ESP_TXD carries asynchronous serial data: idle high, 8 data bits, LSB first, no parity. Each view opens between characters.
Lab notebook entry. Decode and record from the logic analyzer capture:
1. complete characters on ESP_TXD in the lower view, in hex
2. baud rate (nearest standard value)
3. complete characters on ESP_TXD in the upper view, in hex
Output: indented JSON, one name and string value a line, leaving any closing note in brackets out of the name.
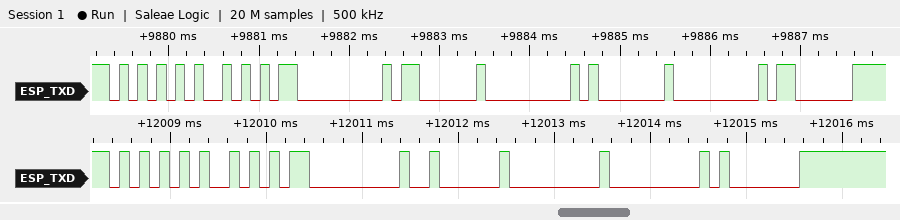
{
  "complete characters on ESP_TXD in the lower view, in hex": "55, AA, 00, 02, 00, 00, 01",
  "baud rate": "9600 baud",
  "complete characters on ESP_TXD in the upper view, in hex": "55, AA, 00, 03, 00, 01, 00, 03"
}
